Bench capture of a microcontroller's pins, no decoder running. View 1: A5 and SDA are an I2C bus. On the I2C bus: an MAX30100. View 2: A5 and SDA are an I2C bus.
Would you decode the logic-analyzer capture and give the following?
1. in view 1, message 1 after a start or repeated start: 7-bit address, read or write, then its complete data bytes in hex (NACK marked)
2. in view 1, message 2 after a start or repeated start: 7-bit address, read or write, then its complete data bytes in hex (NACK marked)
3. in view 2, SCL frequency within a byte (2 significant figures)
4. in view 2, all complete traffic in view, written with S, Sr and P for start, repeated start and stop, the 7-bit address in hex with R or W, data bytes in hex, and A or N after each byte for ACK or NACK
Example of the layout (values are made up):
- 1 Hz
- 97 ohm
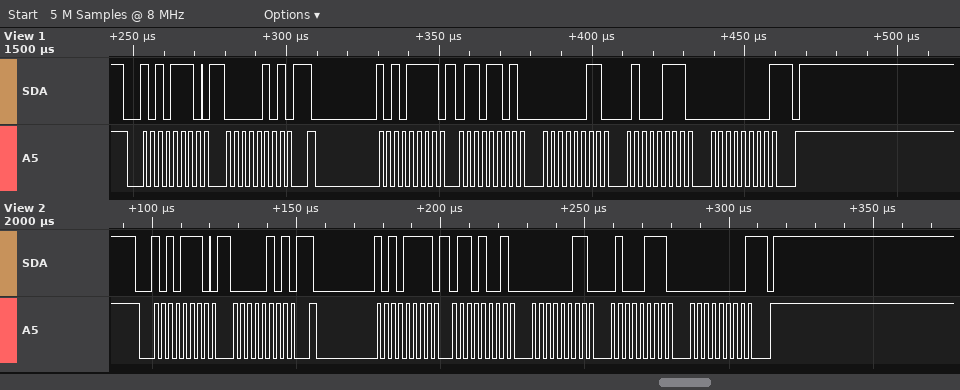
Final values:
- 0x57 write: 05
- 0x57 read: 6D 03 47 00 NACK
- 400 kHz
- S 57W A 05 A Sr 57R A 69 A 03 A 47 A 00 N P
